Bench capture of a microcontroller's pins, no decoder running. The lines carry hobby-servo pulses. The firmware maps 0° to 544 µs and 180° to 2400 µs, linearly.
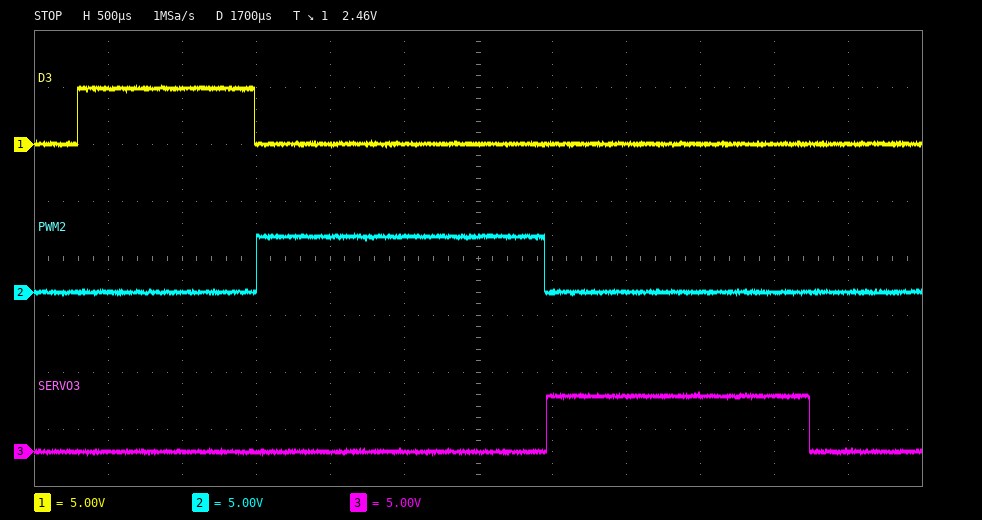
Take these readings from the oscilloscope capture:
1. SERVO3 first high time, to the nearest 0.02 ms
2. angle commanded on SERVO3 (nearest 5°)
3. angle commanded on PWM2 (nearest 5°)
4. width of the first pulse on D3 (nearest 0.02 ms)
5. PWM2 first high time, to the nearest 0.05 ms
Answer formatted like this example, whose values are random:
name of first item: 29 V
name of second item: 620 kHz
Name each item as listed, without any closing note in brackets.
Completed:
SERVO3 first high time, to the nearest 0.02 ms: 1.78 ms
angle commanded on SERVO3: 120°
angle commanded on PWM2: 135°
width of the first pulse on D3: 1.20 ms
PWM2 first high time, to the nearest 0.05 ms: 1.95 ms
